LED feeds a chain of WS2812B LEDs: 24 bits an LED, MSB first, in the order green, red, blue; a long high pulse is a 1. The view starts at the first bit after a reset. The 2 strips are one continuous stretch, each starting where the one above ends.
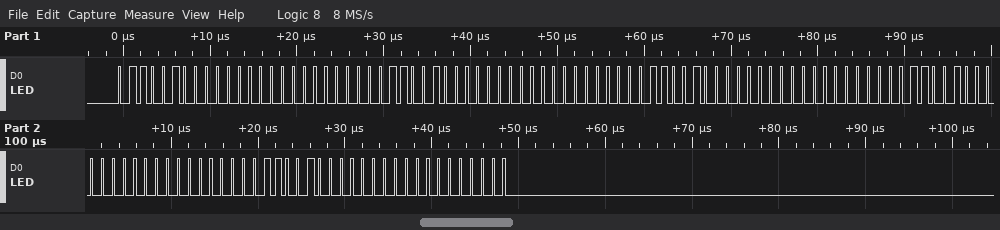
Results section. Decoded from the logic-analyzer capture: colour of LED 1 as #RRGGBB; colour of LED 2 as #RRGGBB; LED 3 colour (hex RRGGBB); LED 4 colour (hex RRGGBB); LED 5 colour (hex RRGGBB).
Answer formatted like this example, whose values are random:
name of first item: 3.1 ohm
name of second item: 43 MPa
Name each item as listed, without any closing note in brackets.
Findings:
colour of LED 1 as #RRGGBB: #006400
colour of LED 2 as #RRGGBB: #006400
LED 3 colour: #006400
LED 4 colour: #006400
LED 5 colour: #006400
